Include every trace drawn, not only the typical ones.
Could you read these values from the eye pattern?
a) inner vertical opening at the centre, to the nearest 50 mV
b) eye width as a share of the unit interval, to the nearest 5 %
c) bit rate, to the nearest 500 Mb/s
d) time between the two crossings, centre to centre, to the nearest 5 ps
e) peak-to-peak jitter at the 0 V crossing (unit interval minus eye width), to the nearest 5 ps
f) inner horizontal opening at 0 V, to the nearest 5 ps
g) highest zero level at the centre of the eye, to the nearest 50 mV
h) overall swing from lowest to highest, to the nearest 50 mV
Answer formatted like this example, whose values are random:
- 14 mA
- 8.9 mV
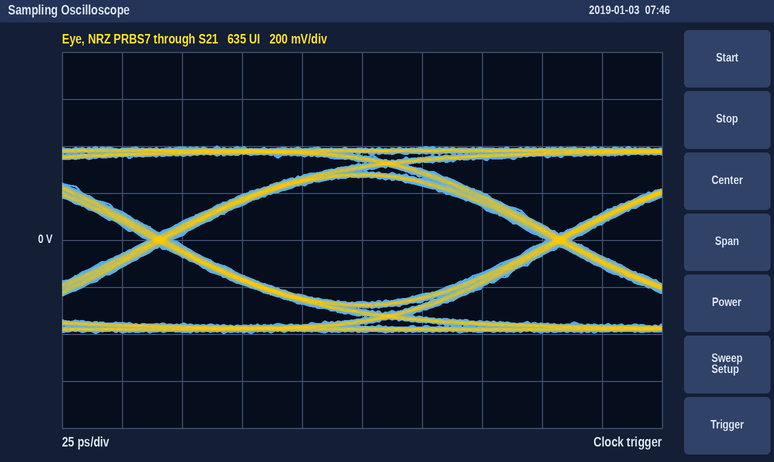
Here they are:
- 550 mV
- 95 %
- 6.0 Gb/s
- 165 ps
- 10 ps
- 155 ps
- -250 mV
- 800 mV
